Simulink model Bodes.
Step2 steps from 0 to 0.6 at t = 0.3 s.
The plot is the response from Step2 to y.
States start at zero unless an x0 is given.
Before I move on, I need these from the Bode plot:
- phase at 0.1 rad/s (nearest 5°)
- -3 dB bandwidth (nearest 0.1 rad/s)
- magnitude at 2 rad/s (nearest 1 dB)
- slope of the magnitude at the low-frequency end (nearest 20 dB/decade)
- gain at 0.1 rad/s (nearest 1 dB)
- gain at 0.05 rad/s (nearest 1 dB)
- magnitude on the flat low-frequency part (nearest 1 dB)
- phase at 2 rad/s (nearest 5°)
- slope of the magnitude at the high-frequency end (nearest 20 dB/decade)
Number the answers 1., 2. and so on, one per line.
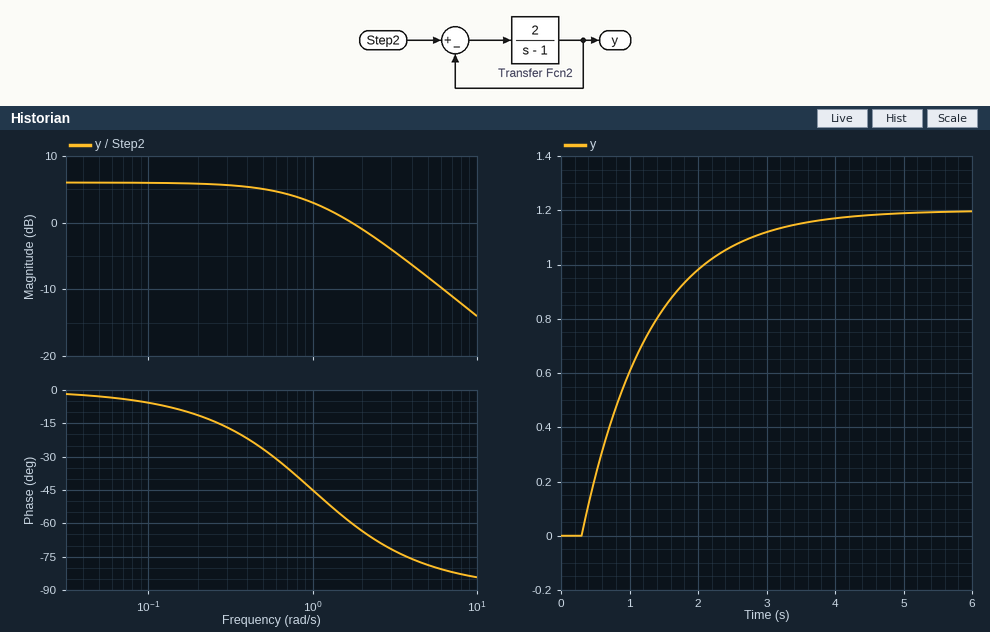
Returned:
1. -5°
2. 1.0 rad/s
3. -1 dB
4. 0 dB/decade
5. 6 dB
6. 6 dB
7. 6 dB
8. -65°
9. -20 dB/decade
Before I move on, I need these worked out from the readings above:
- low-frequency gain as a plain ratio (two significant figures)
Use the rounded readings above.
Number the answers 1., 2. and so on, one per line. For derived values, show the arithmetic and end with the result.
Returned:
1. 10^(6 / 20) = 2.0
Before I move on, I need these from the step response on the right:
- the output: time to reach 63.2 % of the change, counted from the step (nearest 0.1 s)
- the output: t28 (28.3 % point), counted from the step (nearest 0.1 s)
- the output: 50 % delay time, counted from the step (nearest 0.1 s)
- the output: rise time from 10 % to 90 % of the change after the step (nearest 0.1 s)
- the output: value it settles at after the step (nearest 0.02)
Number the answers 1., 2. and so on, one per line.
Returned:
1. 1.0 s
2. 0.3 s
3. 0.7 s
4. 2.2 s
5. 1.20
